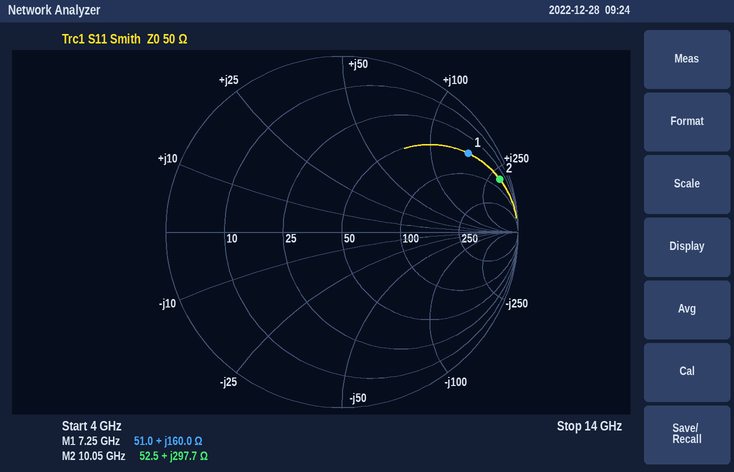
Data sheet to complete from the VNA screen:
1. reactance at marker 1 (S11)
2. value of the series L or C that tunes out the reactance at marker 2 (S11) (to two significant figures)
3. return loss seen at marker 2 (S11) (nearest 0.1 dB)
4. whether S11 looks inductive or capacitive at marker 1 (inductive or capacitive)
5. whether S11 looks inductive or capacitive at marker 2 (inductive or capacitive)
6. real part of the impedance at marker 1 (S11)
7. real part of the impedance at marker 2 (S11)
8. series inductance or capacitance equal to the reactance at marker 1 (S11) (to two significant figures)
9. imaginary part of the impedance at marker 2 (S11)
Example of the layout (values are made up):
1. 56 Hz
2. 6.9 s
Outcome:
1. +160.0 Ω
2. 53 fF
3. 0.5 dB
4. inductive
5. inductive
6. 51.0 Ω
7. 52.5 Ω
8. 3.5 nH
9. +297.7 Ω
